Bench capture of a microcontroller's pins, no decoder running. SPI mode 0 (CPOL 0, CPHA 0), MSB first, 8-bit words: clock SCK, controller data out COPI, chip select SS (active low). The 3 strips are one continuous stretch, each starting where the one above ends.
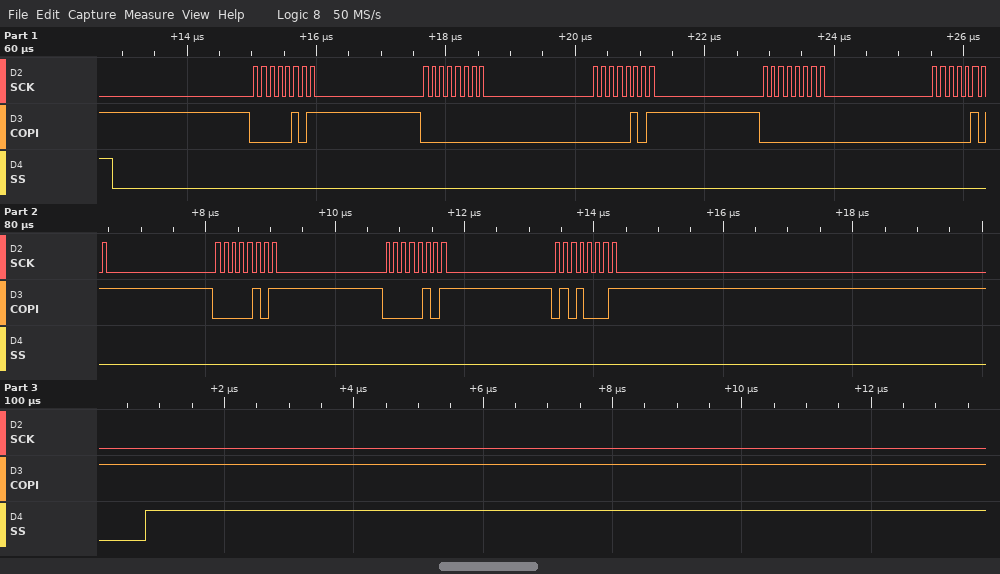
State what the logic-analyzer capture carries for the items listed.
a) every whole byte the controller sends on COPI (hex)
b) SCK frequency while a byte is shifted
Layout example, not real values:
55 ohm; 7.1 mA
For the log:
05 00 05 00 05 05 05 51; 8 MHz
